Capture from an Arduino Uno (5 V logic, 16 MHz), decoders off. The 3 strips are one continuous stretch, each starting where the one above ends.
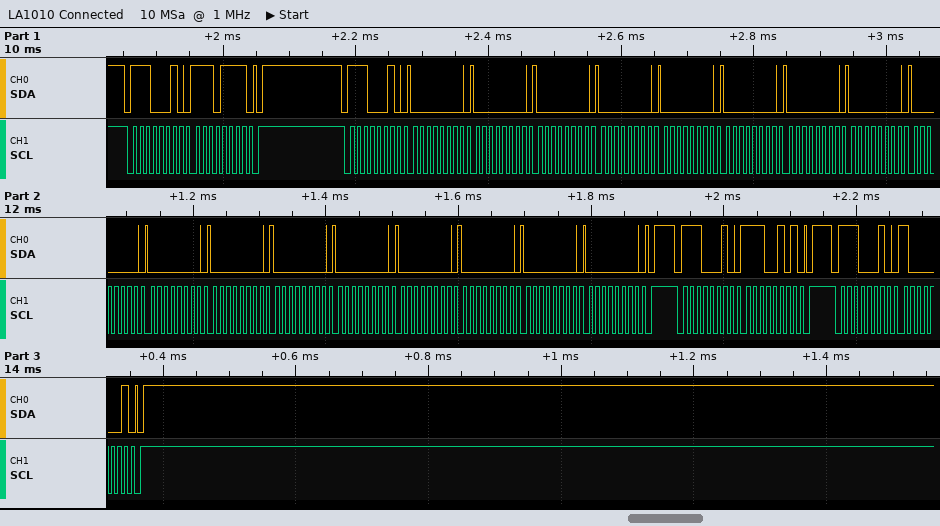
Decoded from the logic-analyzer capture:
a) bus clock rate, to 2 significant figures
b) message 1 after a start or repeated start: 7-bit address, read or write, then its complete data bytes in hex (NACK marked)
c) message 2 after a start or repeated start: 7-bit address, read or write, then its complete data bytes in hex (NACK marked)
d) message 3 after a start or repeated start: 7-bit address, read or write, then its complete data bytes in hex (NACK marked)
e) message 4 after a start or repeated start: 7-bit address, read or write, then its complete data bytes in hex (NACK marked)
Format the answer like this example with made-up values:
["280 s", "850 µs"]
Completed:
["100 kHz", "0x71 write: EF", "0x71 write: 00 00 00 00 00 00 00 00 00 00 00 00 00 00 00 00 00", "0x71 write: E5", "0x71 write: 81"]
